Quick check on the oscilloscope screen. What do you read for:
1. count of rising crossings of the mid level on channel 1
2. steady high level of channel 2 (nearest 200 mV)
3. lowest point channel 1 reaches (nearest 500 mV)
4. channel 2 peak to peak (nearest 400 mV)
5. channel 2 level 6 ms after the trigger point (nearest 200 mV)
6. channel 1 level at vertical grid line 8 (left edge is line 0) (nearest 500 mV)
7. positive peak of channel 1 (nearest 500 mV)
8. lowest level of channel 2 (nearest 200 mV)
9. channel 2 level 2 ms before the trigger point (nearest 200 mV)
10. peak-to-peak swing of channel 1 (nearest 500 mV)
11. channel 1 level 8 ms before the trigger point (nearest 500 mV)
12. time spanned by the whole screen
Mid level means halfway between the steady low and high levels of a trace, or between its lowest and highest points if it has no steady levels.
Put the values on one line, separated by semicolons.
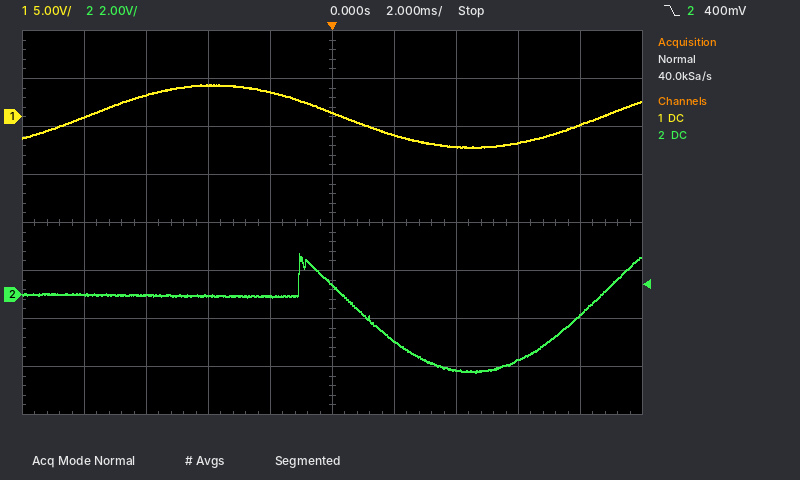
2; 0.0 V; -3.0 V; 4.8 V; -2.8 V; -2.5 V; 3.5 V; -3.2 V; 0.0 V; 6.5 V; 0.0 V; 20 ms
